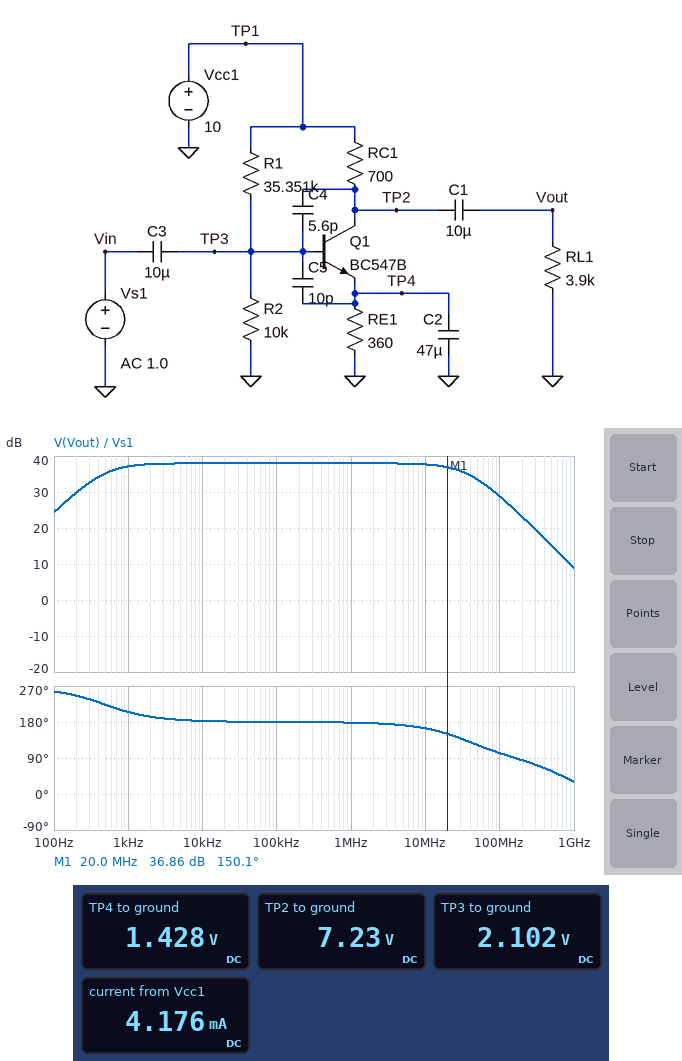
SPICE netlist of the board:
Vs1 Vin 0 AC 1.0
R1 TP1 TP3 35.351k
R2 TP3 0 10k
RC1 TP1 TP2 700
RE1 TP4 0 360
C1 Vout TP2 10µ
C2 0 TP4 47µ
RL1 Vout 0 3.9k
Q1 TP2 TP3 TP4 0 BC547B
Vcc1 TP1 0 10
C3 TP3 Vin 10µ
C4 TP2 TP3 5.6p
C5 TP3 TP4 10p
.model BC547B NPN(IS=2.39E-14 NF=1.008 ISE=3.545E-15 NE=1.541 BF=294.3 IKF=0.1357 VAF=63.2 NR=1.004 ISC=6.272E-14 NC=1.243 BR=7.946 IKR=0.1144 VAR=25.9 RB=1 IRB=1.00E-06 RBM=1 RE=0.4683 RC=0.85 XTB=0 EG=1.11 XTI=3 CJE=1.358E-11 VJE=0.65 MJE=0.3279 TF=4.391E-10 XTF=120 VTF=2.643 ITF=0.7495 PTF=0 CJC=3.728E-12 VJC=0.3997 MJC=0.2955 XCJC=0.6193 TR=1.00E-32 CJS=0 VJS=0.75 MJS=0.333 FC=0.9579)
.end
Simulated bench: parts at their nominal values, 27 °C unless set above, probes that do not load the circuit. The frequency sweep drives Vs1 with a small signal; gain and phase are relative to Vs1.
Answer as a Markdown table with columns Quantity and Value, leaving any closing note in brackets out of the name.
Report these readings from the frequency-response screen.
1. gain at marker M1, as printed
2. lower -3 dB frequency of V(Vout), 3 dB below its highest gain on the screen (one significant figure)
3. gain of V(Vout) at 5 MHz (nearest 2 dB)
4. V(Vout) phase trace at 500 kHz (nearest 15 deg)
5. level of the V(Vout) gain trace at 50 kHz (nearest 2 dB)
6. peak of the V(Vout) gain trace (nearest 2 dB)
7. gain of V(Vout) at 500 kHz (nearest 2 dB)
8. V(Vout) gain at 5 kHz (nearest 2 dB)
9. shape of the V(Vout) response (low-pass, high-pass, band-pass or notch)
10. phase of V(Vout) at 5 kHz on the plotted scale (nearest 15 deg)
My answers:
| Quantity | Value |
|---|---|
| gain at marker M1, as printed | 36.86 dB |
| lower -3 dB frequency of V(Vout), 3 dB below its highest gain on the screen | 500 Hz |
| gain of V(Vout) at 5 MHz | 38 dB |
| V(Vout) phase trace at 500 kHz | 180 deg |
| level of the V(Vout) gain trace at 50 kHz | 38 dB |
| peak of the V(Vout) gain trace | 38 dB |
| gain of V(Vout) at 500 kHz | 38 dB |
| V(Vout) gain at 5 kHz | 38 dB |
| shape of the V(Vout) response | band-pass |
| phase of V(Vout) at 5 kHz on the plotted scale | 180 deg |
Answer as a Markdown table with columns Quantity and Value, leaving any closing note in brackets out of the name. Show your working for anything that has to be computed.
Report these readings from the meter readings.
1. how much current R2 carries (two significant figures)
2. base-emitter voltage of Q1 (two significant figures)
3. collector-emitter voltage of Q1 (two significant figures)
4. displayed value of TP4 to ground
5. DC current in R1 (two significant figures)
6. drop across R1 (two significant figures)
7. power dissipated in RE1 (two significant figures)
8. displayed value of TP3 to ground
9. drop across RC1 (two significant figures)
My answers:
| Quantity | Value |
|---|---|
| how much current R2 carries | (2.102 V) / 10 kΩ = 210 µA |
| base-emitter voltage of Q1 | 2.102 V - 1.428 V = 670 mV |
| collector-emitter voltage of Q1 | 7.23 V - 1.428 V = 5.8 V |
| displayed value of TP4 to ground | 1.428 V |
| DC current in R1 | (10 V - 2.102 V) / 35.35 kΩ = 220 µA |
| drop across R1 | 10 V - 2.102 V = 7.9 V |
| power dissipated in RE1 | (1.428 V)^2 / 360 Ω = 5.7 mW |
| displayed value of TP3 to ground | 2.102 V |
| drop across RC1 | 10 V - 7.23 V = 2.8 V |
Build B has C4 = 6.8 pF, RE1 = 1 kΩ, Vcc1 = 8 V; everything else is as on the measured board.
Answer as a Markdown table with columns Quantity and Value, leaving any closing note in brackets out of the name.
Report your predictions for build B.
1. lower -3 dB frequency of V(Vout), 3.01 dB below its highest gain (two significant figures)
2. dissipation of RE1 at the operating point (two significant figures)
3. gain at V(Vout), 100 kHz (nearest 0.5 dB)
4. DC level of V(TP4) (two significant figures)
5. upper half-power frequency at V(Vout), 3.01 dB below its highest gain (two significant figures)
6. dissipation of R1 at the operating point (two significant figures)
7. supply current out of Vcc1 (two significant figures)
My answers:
| Quantity | Value |
|---|---|
| lower -3 dB frequency of V(Vout), 3.01 dB below its highest gain | 140 Hz |
| dissipation of RE1 at the operating point | 1.2 mW |
| gain at V(Vout), 100 kHz | 27.5 dB |
| DC level of V(TP4) | 1.1 V |
| upper half-power frequency at V(Vout), 3.01 dB below its highest gain | 32 MHz |
| dissipation of R1 at the operating point | 1.1 mW |
| supply current out of Vcc1 | 1.3 mA |
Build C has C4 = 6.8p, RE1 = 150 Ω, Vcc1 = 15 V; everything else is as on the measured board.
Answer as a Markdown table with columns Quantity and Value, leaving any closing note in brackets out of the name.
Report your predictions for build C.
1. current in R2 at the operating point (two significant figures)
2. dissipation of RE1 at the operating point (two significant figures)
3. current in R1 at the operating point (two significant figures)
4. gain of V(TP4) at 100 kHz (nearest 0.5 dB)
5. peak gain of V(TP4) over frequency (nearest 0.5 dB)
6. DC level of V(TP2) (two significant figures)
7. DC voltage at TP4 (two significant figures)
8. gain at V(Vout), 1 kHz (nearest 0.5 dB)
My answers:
| Quantity | Value |
|---|---|
| current in R2 at the operating point | 290 µA |
| dissipation of RE1 at the operating point | 31 mW |
| current in R1 at the operating point | 340 µA |
| gain of V(TP4) at 100 kHz | -38.0 dB |
| peak gain of V(TP4) over frequency | -0.5 dB |
| DC level of V(TP2) | 4.9 V |
| DC voltage at TP4 | 2.2 V |
| gain at V(Vout), 1 kHz | 42.5 dB |
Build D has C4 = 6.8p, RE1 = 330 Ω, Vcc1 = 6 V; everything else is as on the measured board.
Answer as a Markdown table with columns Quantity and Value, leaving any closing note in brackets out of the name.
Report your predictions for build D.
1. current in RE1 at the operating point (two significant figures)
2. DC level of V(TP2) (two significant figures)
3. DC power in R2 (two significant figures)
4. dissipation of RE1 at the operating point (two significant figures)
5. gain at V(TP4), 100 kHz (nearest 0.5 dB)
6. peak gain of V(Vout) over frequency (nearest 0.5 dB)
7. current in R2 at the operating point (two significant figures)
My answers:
| Quantity | Value |
|---|---|
| current in RE1 at the operating point | 1.9 mA |
| DC level of V(TP2) | 4.7 V |
| DC power in R2 | 160 µW |
| dissipation of RE1 at the operating point | 1.2 mW |
| gain at V(TP4), 100 kHz | -53.0 dB |
| peak gain of V(Vout) over frequency | 32.0 dB |
| current in R2 at the operating point | 130 µA |
